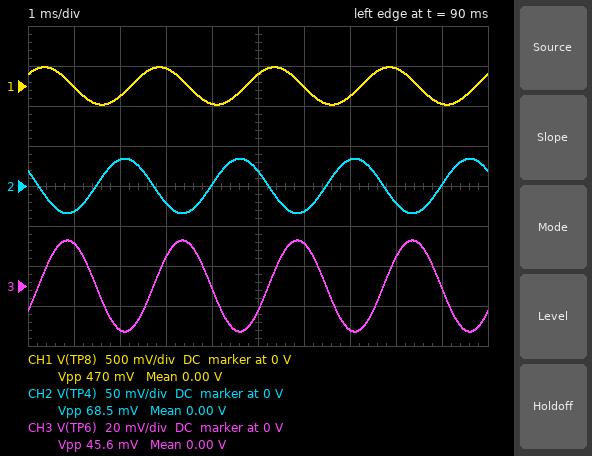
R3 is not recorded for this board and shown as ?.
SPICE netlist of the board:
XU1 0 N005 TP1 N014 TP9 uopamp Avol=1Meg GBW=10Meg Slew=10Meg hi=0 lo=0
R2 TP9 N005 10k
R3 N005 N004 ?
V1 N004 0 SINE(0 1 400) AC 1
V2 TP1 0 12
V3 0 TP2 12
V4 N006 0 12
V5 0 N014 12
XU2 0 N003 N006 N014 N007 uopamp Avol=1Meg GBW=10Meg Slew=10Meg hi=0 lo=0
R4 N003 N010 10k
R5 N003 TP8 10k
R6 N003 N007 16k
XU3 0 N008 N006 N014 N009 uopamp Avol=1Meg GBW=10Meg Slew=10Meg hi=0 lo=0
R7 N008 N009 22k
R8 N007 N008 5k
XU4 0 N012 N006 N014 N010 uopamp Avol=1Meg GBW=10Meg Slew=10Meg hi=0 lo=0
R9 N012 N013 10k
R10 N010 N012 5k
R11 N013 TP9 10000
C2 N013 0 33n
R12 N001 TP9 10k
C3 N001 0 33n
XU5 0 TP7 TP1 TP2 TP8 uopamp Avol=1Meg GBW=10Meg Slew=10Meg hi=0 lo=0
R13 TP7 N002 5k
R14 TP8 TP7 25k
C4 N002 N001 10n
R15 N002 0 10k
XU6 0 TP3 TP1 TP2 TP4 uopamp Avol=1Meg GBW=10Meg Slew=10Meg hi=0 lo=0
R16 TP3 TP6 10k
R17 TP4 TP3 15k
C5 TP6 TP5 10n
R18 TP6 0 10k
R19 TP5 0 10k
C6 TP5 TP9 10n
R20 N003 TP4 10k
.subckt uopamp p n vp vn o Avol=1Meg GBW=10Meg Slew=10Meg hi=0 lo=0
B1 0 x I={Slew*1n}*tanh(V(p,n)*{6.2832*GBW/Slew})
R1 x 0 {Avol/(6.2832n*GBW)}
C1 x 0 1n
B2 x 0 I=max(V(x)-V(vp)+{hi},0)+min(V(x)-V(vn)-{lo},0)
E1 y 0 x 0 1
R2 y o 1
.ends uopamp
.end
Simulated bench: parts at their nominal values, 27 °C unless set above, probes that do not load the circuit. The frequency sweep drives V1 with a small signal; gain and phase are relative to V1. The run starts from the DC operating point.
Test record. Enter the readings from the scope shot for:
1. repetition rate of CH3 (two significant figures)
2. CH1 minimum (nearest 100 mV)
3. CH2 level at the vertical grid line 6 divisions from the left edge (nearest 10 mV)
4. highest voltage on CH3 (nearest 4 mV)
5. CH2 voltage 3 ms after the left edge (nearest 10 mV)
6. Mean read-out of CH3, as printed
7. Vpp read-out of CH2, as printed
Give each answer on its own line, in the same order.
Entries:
400 Hz
-200 mV
-30 mV
24 mV
-20 mV
0.00 V
68.5 mV
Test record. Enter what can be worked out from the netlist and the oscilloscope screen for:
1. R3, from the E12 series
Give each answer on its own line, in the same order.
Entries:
12 kΩ
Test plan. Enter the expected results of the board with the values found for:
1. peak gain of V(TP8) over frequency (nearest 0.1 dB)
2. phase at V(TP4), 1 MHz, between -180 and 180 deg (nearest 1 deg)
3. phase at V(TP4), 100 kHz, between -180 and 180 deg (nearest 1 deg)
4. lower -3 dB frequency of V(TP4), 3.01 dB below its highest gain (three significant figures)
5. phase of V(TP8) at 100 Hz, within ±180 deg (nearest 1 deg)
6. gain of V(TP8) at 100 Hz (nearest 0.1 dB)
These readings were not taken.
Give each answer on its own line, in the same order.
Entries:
-10.5 dB
-24 deg
2 deg
7.30 kHz
74 deg
-21.5 dB
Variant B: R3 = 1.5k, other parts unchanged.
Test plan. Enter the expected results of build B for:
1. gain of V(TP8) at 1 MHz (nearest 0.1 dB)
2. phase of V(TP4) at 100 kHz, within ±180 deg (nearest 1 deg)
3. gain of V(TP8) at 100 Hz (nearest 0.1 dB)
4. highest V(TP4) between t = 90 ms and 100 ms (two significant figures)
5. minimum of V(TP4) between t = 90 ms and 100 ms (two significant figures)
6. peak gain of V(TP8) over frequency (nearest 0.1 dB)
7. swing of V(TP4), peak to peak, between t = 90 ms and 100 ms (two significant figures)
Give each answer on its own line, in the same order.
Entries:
-39.2 dB
-1 deg
-3.4 dB
270 mV
-270 mV
7.6 dB
550 mV
